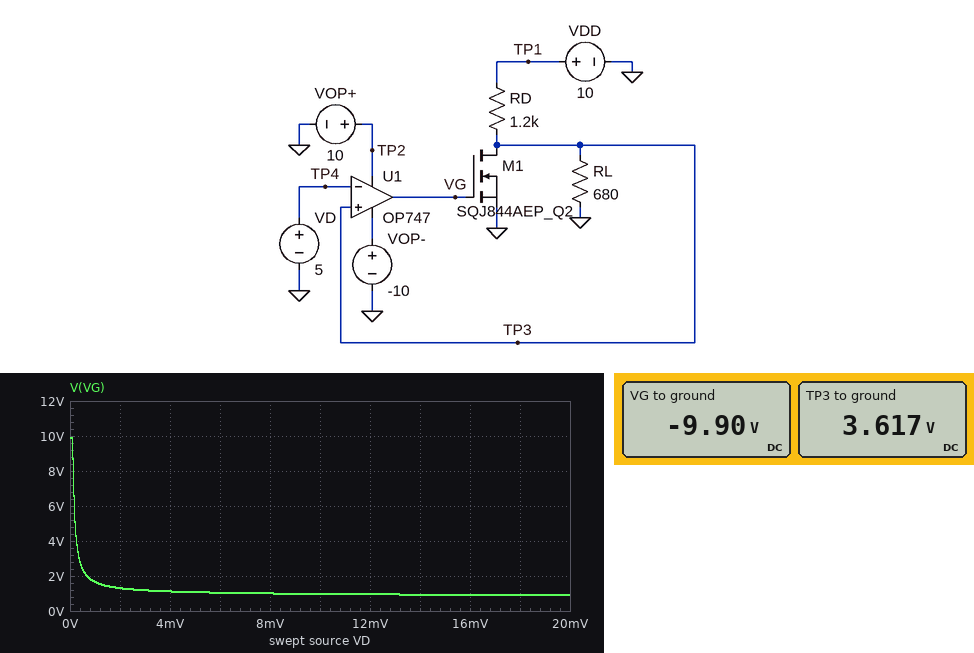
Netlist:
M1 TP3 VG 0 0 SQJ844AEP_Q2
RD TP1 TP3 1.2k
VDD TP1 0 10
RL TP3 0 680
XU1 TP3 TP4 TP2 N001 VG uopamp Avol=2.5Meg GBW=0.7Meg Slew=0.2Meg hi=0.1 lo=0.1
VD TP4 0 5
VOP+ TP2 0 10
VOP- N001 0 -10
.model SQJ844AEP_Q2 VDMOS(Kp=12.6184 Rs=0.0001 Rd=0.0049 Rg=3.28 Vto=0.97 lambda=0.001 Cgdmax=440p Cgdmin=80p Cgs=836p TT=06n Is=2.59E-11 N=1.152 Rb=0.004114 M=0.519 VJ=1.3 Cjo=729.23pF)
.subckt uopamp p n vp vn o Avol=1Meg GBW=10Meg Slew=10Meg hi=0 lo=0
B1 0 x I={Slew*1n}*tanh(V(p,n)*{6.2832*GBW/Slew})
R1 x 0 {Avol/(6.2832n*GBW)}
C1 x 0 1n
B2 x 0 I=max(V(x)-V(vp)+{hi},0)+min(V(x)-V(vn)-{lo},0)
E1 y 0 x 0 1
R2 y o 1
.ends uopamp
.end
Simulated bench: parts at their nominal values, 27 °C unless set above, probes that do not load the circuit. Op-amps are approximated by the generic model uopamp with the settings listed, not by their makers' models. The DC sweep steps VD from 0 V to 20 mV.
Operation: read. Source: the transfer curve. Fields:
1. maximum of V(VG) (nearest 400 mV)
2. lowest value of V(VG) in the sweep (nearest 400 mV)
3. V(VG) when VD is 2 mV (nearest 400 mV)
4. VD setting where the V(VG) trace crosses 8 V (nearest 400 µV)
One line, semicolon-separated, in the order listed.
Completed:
10.0 V; 800 mV; 1.2 V; 0 V
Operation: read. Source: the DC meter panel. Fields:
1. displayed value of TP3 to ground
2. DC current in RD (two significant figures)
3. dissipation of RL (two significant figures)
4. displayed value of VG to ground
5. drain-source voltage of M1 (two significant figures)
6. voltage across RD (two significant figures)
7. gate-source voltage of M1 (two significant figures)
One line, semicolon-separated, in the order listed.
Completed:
3.617 V; 5.3 mA; 19 mW; -9.90 V; 3.6 V; 6.4 V; -9.9 V
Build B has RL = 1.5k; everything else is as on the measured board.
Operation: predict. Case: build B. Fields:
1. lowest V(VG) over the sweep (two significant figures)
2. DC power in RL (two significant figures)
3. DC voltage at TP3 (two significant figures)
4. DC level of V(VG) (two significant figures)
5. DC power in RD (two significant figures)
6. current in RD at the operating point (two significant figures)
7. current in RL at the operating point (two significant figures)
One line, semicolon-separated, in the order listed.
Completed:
910 mV; 17 mW; 5.0 V; 760 mV; 21 mW; 4.2 mA; 3.3 mA
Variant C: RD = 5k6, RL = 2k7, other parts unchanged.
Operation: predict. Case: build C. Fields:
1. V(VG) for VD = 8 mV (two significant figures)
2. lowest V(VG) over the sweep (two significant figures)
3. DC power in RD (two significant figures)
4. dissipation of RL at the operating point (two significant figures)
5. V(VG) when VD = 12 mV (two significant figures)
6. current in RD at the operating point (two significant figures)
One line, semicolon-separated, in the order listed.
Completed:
830 mV; 800 mV; 8.1 mW; 3.9 mW; 810 mV; 1.2 mA
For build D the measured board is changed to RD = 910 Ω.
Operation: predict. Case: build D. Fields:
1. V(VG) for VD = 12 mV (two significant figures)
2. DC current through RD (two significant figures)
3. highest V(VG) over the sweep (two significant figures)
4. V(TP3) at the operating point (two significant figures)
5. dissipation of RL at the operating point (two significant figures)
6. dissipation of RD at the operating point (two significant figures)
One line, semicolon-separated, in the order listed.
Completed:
990 mV; 6.3 mA; 9.9 V; 4.3 V; 27 mW; 36 mW
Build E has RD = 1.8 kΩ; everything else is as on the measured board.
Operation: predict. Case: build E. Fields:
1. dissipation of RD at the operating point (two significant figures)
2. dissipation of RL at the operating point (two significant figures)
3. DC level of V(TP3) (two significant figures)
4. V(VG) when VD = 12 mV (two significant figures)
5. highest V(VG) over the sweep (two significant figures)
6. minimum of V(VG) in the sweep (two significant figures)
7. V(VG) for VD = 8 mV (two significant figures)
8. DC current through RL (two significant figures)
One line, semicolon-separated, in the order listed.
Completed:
29 mW; 11 mW; 2.7 V; 910 mV; 9.9 V; 870 mV; 950 mV; 4.0 mA
